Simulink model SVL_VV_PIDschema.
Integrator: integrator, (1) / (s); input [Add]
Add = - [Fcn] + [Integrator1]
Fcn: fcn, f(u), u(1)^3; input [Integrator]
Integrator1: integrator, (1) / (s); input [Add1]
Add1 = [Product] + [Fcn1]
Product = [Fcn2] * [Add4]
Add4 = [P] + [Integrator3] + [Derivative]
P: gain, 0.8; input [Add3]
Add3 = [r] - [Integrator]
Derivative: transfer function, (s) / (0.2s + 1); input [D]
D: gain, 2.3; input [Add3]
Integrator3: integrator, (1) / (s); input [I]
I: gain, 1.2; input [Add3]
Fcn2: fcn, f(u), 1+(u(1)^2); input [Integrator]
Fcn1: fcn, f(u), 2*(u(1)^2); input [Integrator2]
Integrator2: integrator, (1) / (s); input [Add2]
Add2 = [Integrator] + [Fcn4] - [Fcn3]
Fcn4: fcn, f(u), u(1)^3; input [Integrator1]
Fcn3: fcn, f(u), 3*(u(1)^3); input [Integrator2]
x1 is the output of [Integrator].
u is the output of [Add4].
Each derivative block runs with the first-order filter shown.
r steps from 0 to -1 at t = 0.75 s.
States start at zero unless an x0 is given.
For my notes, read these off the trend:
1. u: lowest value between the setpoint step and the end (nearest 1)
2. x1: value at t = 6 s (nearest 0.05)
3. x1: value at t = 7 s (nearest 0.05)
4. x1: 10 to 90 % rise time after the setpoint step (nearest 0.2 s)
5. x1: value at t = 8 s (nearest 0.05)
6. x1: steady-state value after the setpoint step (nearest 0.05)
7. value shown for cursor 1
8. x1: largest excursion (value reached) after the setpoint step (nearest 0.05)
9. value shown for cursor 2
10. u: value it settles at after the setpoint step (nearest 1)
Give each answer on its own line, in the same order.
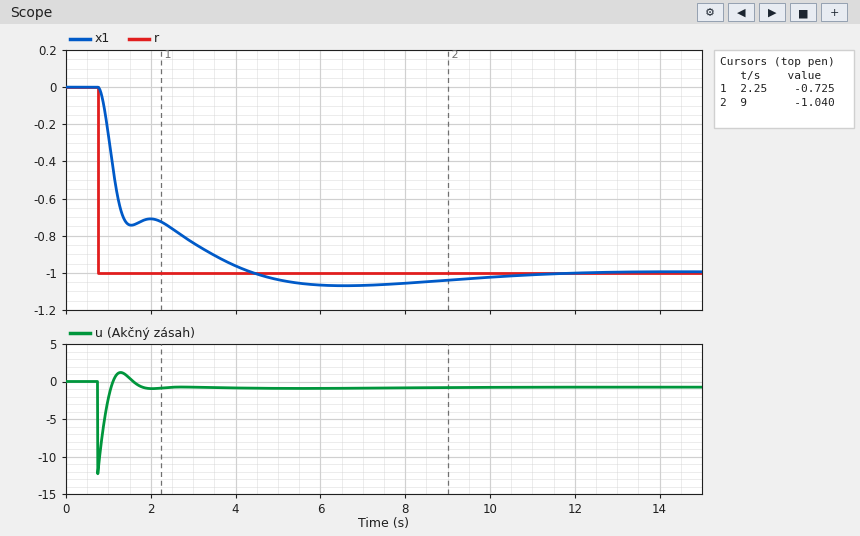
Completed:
-12
-1.05
-1.05
2.6 s
-1.05
-1.00
-0.725
-1.05
-1.040
-1
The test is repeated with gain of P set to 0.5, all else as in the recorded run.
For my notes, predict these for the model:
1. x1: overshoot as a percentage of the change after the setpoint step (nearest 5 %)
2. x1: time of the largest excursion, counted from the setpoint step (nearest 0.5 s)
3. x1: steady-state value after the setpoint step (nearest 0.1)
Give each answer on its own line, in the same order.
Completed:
10 %
6.0 s
-1.0
